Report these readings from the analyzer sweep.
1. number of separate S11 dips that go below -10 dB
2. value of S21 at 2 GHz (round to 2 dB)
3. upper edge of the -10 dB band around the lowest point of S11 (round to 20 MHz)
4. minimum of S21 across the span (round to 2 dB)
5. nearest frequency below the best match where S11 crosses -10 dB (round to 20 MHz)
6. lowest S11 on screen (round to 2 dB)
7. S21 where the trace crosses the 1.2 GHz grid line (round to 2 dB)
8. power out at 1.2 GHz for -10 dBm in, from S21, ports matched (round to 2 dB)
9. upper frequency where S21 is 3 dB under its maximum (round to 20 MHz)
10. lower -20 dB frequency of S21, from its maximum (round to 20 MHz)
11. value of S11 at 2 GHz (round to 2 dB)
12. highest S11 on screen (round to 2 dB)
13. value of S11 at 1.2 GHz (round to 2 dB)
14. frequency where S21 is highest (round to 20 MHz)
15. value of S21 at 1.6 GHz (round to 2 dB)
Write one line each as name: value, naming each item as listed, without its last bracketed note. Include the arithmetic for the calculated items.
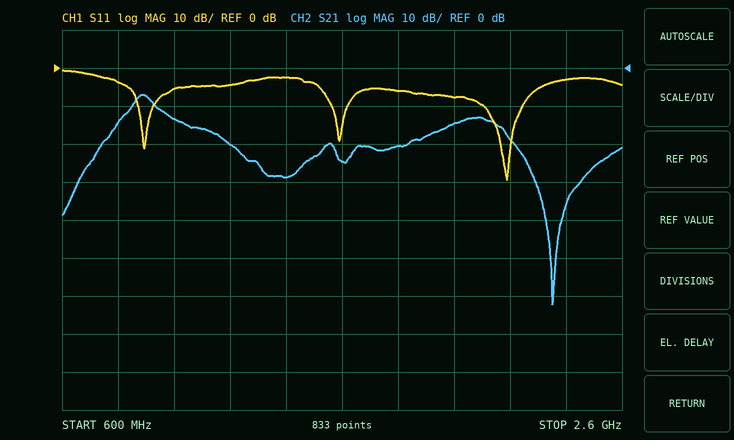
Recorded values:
number of separate S11 dips that go below -10 dB: 3
value of S21 at 2 GHz: -14 dB
upper edge of the -10 dB band around the lowest point of S11: 2.24 GHz
minimum of S21 across the span: -62 dB
nearest frequency below the best match where S11 crosses -10 dB: 2.10 GHz
lowest S11 on screen: -30 dB
S21 where the trace crosses the 1.2 GHz grid line: -20 dB
power out at 1.2 GHz for -10 dBm in, from S21, ports matched: -10 dBm + (-20 dB) = -30 dBm
upper frequency where S21 is 3 dB under its maximum: 940 MHz
lower -20 dB frequency of S21, from its maximum: 680 MHz
value of S11 at 2 GHz: -8 dB
highest S11 on screen: 0 dB
value of S11 at 1.2 GHz: -4 dB
frequency where S21 is highest: 880 MHz
value of S21 at 1.6 GHz: -24 dB
